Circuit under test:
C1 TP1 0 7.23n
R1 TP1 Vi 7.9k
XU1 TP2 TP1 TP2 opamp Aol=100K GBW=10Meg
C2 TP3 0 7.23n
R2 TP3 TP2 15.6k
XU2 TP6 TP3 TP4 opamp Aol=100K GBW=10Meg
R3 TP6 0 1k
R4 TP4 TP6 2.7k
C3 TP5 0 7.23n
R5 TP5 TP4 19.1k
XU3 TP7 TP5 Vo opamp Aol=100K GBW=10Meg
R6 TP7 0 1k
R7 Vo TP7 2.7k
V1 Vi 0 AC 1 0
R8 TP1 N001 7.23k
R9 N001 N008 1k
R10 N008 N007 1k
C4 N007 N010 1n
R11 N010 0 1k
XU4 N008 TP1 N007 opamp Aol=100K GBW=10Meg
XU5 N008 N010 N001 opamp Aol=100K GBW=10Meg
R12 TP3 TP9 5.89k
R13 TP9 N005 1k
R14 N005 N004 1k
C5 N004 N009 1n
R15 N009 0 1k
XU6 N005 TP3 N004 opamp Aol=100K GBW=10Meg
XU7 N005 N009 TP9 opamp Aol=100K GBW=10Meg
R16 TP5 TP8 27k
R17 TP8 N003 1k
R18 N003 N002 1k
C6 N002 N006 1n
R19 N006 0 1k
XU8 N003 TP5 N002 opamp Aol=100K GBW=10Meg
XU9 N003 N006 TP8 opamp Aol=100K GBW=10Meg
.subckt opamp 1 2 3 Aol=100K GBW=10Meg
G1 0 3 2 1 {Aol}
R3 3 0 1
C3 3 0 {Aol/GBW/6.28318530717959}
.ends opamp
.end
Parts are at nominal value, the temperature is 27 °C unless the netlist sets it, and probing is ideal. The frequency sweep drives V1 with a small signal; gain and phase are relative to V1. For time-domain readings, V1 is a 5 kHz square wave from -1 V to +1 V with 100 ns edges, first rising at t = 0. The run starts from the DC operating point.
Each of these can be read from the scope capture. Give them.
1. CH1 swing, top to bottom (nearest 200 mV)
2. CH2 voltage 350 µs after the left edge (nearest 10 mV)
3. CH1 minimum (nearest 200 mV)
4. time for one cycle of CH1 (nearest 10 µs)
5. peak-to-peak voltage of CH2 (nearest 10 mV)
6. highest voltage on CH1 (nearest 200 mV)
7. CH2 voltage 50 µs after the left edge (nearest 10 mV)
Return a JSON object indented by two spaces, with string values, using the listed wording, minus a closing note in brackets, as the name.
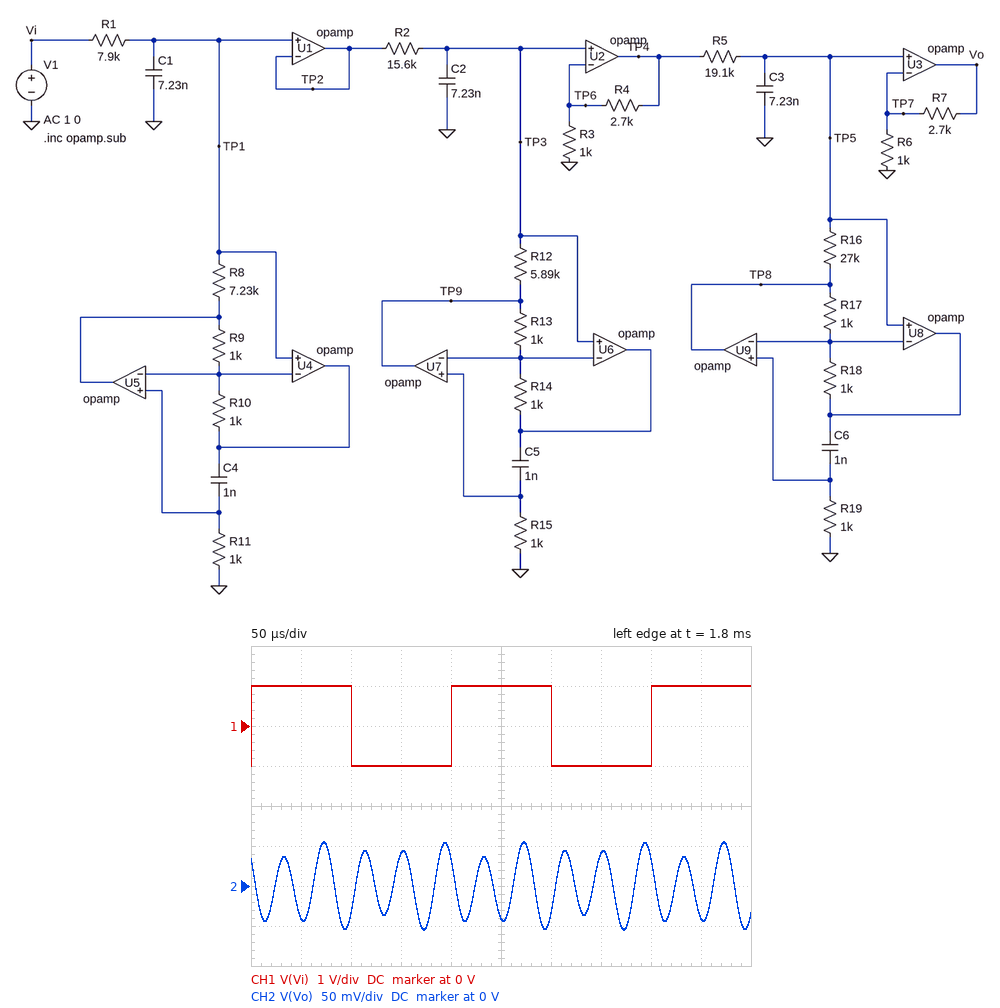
{
  "CH1 swing, top to bottom": "2.0 V",
  "CH2 voltage 350 µs after the left edge": "40 mV",
  "CH1 minimum": "-1.0 V",
  "time for one cycle of CH1": "200 µs",
  "peak-to-peak voltage of CH2": "110 mV",
  "highest voltage on CH1": "1.0 V",
  "CH2 voltage 50 µs after the left edge": "-40 mV"
}
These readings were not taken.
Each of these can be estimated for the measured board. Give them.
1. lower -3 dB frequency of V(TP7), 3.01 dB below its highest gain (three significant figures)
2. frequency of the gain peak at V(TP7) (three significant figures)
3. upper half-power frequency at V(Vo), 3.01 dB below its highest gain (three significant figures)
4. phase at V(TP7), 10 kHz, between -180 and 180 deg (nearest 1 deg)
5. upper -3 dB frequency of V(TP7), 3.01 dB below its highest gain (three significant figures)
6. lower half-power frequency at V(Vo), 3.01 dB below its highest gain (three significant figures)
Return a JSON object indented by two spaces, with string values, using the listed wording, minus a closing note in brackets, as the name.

{
  "lower -3 dB frequency of V(TP7), 3.01 dB below its highest gain": "22.4 kHz",
  "frequency of the gain peak at V(TP7)": "23.8 kHz",
  "upper half-power frequency at V(Vo), 3.01 dB below its highest gain": "24.4 kHz",
  "phase at V(TP7), 10 kHz, between -180 and 180 deg": "-121 deg",
  "upper -3 dB frequency of V(TP7), 3.01 dB below its highest gain": "24.4 kHz",
  "lower half-power frequency at V(Vo), 3.01 dB below its highest gain": "22.4 kHz"
}
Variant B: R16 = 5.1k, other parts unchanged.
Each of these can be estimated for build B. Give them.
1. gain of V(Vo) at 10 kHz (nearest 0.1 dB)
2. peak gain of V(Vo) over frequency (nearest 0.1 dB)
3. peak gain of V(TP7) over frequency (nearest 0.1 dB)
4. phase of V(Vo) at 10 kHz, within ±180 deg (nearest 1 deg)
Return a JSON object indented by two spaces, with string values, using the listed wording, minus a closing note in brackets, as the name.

{
  "gain of V(Vo) at 10 kHz": "-64.1 dB",
  "peak gain of V(Vo) over frequency": "6.8 dB",
  "peak gain of V(TP7) over frequency": "-4.6 dB",
  "phase of V(Vo) at 10 kHz, within ±180 deg": "-98 deg"
}
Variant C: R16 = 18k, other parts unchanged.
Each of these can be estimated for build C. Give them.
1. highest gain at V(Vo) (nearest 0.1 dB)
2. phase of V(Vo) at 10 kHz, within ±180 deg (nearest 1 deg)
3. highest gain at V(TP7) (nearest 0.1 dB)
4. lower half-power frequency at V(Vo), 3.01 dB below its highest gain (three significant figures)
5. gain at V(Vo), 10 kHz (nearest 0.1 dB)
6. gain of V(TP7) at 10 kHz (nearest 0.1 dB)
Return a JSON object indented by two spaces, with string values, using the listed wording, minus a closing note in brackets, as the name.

{
  "highest gain at V(Vo)": "-5.4 dB",
  "phase of V(Vo) at 10 kHz, within ±180 deg": "-104 deg",
  "highest gain at V(TP7)": "-16.8 dB",
  "lower half-power frequency at V(Vo), 3.01 dB below its highest gain": "22.2 kHz",
  "gain at V(Vo), 10 kHz": "-48.1 dB",
  "gain of V(TP7) at 10 kHz": "-59.5 dB"
}
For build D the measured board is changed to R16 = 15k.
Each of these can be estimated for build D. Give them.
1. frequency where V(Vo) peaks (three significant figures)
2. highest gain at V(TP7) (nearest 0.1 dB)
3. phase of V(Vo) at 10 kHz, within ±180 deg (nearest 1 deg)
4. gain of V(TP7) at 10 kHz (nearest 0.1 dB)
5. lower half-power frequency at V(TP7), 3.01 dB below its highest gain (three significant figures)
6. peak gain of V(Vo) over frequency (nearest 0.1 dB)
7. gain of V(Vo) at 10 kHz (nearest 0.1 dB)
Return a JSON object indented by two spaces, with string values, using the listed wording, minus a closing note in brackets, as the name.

{
  "frequency where V(Vo) peaks": "23.8 kHz",
  "highest gain at V(TP7)": "-15.9 dB",
  "phase of V(Vo) at 10 kHz, within ±180 deg": "-102 deg",
  "gain of V(TP7) at 10 kHz": "-62.5 dB",
  "lower half-power frequency at V(TP7), 3.01 dB below its highest gain": "22.1 kHz",
  "peak gain of V(Vo) over frequency": "-4.5 dB",
  "gain of V(Vo) at 10 kHz": "-51.2 dB"
}
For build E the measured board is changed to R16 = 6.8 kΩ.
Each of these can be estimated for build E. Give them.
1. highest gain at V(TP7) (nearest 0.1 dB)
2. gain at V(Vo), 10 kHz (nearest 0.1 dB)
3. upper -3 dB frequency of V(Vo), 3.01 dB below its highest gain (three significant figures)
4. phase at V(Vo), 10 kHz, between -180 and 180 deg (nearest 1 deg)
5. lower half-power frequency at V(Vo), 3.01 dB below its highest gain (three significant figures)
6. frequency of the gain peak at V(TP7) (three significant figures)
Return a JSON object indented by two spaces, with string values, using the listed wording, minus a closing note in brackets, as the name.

{
  "highest gain at V(TP7)": "2.1 dB",
  "gain at V(Vo), 10 kHz": "-61.1 dB",
  "upper -3 dB frequency of V(Vo), 3.01 dB below its highest gain": "23.3 kHz",
  "phase at V(Vo), 10 kHz, between -180 and 180 deg": "-98 deg",
  "lower half-power frequency at V(Vo), 3.01 dB below its highest gain": "21.9 kHz",
  "frequency of the gain peak at V(TP7)": "22.4 kHz"
}
